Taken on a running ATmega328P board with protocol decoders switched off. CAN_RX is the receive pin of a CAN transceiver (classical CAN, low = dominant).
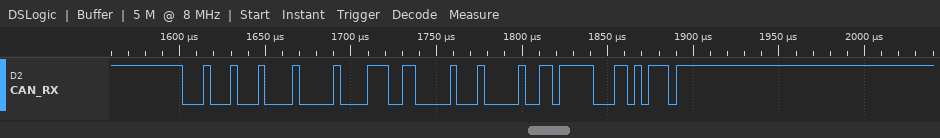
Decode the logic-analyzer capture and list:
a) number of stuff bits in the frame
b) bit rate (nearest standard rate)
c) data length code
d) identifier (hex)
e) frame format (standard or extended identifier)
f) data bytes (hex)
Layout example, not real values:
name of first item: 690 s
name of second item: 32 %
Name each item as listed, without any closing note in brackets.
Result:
number of stuff bits in the frame: 4
bit rate: 250 kbit/s
data length code: 4
identifier: 0x111
frame format: standard
data bytes: 01 CC 02 03
